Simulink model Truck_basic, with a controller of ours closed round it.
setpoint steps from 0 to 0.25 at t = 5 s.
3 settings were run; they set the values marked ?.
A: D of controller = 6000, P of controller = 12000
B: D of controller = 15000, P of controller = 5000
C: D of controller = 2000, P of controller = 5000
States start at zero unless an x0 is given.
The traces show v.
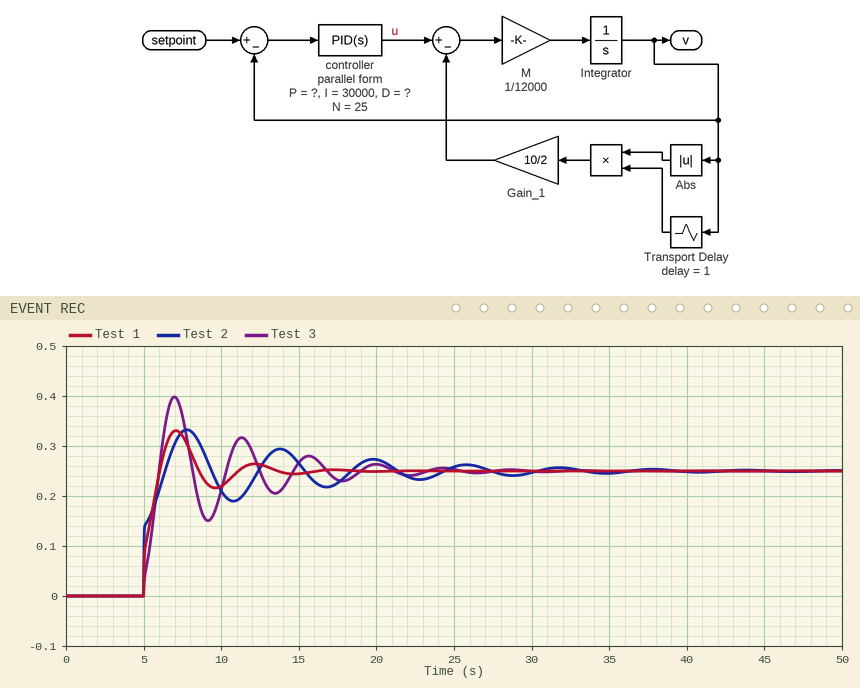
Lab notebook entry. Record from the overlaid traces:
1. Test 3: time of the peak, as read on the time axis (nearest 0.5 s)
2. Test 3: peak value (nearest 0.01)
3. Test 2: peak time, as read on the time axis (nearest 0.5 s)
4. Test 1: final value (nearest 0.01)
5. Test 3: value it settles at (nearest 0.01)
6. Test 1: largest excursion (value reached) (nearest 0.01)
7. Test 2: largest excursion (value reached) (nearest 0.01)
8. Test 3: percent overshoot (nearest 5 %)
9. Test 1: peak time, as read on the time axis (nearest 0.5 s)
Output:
7.0 s
0.40
8.0 s
0.25
0.25
0.33
0.33
60 %
7.0 s
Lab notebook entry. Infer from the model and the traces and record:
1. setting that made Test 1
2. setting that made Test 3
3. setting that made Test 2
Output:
A
C
B
